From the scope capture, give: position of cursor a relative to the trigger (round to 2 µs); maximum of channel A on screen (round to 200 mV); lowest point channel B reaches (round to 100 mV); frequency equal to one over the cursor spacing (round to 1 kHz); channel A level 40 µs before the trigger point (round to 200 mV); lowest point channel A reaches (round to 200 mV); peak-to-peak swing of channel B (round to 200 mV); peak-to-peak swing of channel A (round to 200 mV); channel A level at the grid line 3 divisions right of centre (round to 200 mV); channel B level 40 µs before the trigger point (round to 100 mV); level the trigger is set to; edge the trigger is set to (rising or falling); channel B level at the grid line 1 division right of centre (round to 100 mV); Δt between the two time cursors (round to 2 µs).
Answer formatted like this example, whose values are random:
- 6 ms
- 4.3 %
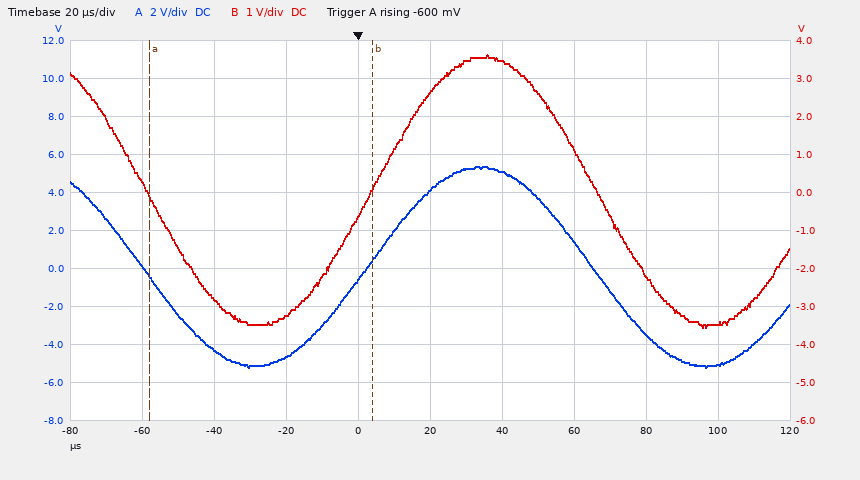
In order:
- -58 µs
- 5.4 V
- -3.6 V
- 16 kHz
- -4.2 V
- -5.2 V
- 7.2 V
- 10.6 V
- -3.4 V
- -2.8 V
- -600 mV
- rising
- 3.4 V
- 62 µs
